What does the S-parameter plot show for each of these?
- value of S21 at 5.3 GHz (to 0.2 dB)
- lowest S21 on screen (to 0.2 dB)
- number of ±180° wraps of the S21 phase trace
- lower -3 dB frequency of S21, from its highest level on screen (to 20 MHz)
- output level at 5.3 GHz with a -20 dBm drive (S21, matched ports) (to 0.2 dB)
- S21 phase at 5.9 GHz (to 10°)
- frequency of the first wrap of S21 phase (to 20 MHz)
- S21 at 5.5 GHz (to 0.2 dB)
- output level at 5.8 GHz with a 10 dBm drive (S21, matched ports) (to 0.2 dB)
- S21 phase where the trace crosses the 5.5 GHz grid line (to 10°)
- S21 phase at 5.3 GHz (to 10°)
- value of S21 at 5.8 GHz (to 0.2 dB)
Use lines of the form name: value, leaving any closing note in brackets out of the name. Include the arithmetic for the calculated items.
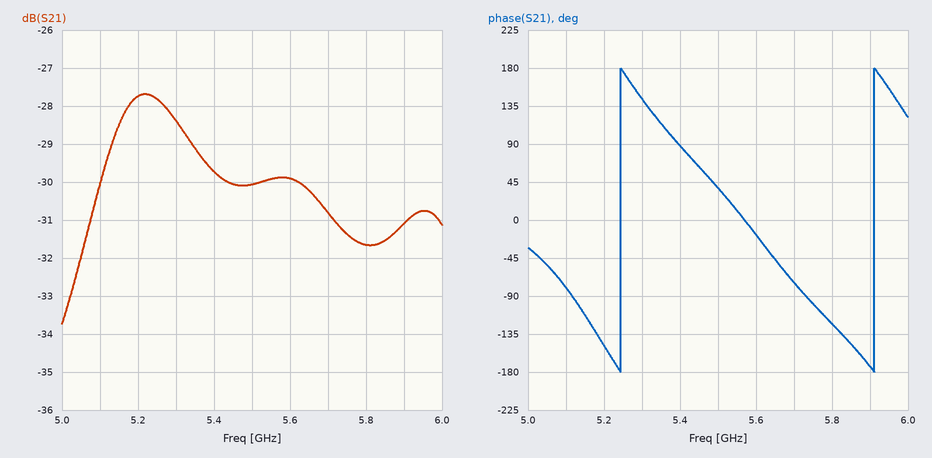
value of S21 at 5.3 GHz: -28.4 dB
lowest S21 on screen: -33.8 dB
number of ±180° wraps of the S21 phase trace: 2
lower -3 dB frequency of S21, from its highest level on screen: 5.08 GHz
output level at 5.3 GHz with a -20 dBm drive (S21, matched ports): -20 dBm + (-28.4 dB) = -48.4 dBm
S21 phase at 5.9 GHz: -170°
frequency of the first wrap of S21 phase: 5.24 GHz
S21 at 5.5 GHz: -30.0 dB
output level at 5.8 GHz with a 10 dBm drive (S21, matched ports): 10 dBm + (-31.6 dB) = -21.6 dBm
S21 phase where the trace crosses the 5.5 GHz grid line: 40°
S21 phase at 5.3 GHz: 140°
value of S21 at 5.8 GHz: -31.6 dB
